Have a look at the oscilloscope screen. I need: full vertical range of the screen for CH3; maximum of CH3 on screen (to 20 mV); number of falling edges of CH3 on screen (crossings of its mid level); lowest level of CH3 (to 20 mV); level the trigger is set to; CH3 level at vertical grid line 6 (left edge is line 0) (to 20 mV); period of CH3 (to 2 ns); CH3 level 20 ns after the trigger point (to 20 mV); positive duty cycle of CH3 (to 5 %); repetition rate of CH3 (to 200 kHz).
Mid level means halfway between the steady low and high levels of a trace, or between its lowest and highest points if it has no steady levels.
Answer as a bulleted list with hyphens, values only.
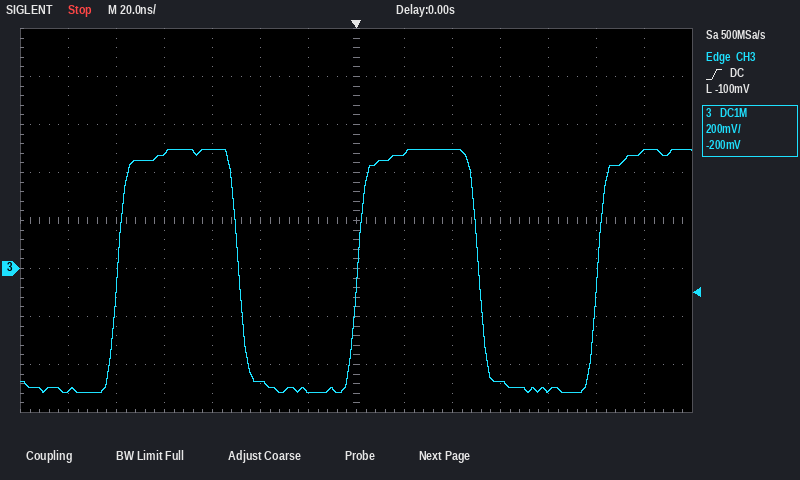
- 1.6 V
- 500 mV
- 2
- -520 mV
- -100 mV
- -520 mV
- 100 ns
- 480 mV
- 50 %
- 10.0 MHz
